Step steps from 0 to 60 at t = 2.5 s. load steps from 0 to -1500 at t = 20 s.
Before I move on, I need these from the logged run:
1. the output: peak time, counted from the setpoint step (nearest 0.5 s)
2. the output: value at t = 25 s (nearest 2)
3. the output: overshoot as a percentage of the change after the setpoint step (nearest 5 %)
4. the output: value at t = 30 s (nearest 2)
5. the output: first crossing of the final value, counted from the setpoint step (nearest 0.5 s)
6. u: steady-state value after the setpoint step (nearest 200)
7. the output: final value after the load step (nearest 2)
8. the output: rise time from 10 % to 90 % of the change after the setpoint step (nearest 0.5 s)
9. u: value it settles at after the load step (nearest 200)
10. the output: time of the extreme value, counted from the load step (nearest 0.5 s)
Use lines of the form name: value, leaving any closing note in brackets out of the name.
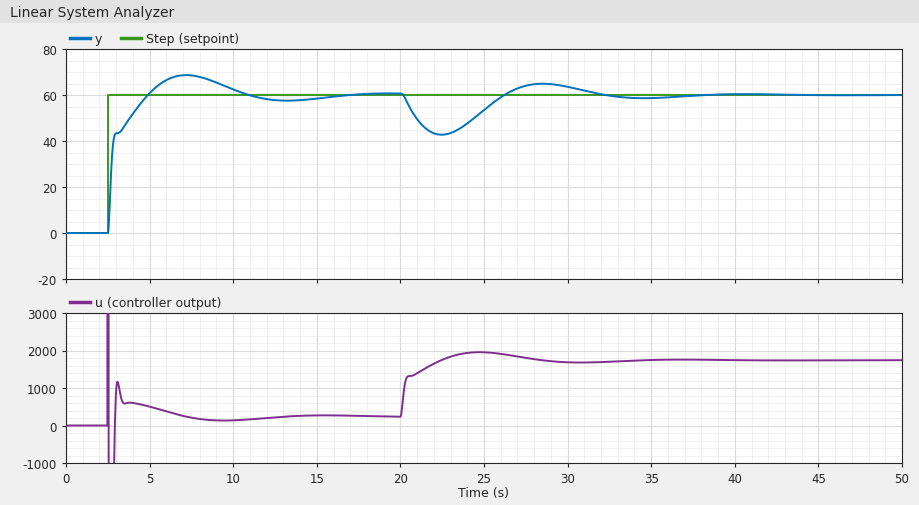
the output: peak time, counted from the setpoint step: 4.5 s
the output: value at t = 25 s: 54
the output: overshoot as a percentage of the change after the setpoint step: 15 %
the output: value at t = 30 s: 64
the output: first crossing of the final value, counted from the setpoint step: 2.5 s
u: steady-state value after the setpoint step: 200
the output: final value after the load step: 60
the output: rise time from 10 % to 90 % of the change after the setpoint step: 1.5 s
u: value it settles at after the load step: 1800
the output: time of the extreme value, counted from the load step: 2.5 s
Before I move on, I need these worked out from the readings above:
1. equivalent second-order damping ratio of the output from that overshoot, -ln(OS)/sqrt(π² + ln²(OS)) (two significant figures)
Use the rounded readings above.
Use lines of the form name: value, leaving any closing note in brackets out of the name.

equivalent second-order damping ratio of the output from that overshoot, -ln(OS)/sqrt(π² + ln²(OS)): 0.52
